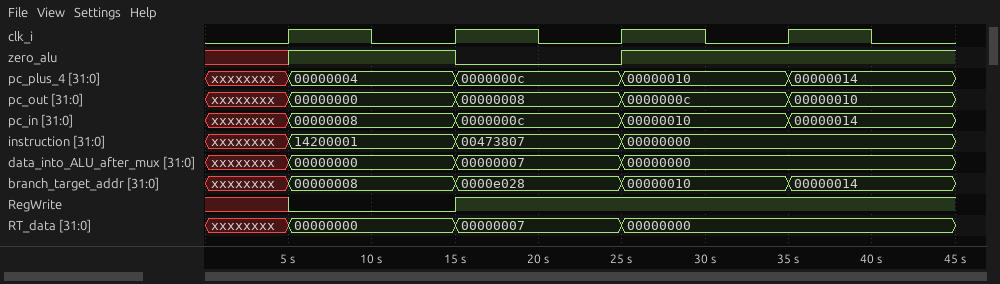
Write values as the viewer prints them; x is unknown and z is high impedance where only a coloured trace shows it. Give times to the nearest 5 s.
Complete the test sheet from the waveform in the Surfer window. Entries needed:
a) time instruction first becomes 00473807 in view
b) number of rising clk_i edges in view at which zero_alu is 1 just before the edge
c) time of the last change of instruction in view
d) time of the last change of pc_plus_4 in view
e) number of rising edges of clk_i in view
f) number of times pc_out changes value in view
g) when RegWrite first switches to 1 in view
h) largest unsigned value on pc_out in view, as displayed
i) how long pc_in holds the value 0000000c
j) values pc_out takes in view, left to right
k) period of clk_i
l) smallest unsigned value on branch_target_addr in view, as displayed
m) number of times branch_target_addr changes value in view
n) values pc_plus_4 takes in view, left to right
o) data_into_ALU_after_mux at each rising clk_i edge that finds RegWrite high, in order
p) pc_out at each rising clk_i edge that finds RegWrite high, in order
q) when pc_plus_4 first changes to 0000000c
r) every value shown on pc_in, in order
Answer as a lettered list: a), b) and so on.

a) 15 s
b) 2
c) 25 s
d) 35 s
e) 4
f) 4
g) 15 s
h) 00000010
i) 10 s
j) xxxxxxxx, 00000000, 00000008, 0000000c, 00000010
k) 10 s
l) 00000008
m) 4
n) xxxxxxxx, 00000004, 0000000c, 00000010, 00000014
o) 00000007, 00000000
p) 00000008, 0000000c
q) 15 s
r) xxxxxxxx, 00000008, 0000000c, 00000010, 00000014
